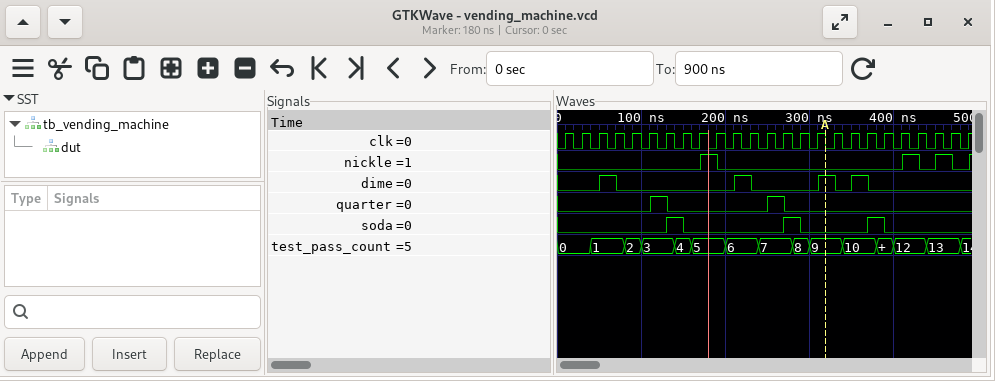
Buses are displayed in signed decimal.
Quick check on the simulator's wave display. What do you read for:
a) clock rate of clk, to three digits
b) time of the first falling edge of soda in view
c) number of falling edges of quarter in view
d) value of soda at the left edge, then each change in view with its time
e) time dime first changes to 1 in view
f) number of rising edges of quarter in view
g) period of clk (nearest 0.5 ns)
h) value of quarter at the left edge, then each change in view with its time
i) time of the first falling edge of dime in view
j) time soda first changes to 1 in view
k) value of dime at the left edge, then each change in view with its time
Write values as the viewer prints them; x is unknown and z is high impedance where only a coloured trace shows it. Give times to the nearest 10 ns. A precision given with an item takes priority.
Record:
50.0 MHz
150 ns
2
0, 1 at 130 ns, 0 at 150 ns, 1 at 270 ns, 0 at 290 ns, 1 at 370 ns, 0 at 390 ns
50 ns
2
20 ns
0, 1 at 110 ns, 0 at 130 ns, 1 at 250 ns, 0 at 270 ns
70 ns
130 ns
0, 1 at 50 ns, 0 at 70 ns, 1 at 210 ns, 0 at 230 ns, 1 at 310 ns, 0 at 330 ns, 1 at 350 ns, 0 at 370 ns
